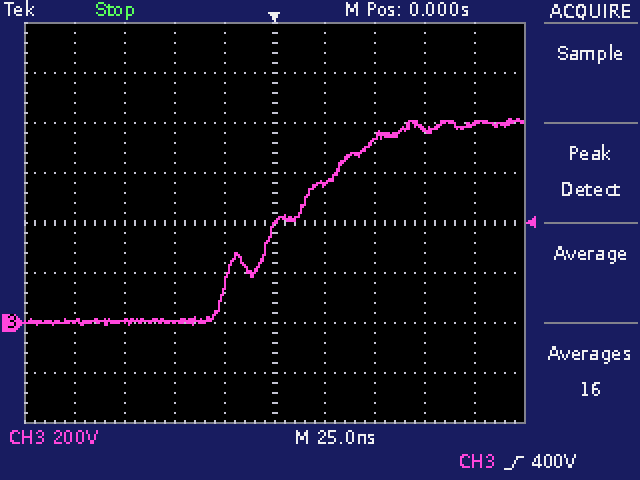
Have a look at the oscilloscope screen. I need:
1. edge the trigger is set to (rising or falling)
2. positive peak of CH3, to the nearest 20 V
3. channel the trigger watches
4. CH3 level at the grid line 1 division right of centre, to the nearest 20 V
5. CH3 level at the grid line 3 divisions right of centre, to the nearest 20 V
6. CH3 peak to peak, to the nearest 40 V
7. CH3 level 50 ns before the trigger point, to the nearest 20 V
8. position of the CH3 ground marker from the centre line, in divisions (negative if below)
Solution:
rising
820 V
CH3
560 V
780 V
840 V
0 V
-2.0 div
